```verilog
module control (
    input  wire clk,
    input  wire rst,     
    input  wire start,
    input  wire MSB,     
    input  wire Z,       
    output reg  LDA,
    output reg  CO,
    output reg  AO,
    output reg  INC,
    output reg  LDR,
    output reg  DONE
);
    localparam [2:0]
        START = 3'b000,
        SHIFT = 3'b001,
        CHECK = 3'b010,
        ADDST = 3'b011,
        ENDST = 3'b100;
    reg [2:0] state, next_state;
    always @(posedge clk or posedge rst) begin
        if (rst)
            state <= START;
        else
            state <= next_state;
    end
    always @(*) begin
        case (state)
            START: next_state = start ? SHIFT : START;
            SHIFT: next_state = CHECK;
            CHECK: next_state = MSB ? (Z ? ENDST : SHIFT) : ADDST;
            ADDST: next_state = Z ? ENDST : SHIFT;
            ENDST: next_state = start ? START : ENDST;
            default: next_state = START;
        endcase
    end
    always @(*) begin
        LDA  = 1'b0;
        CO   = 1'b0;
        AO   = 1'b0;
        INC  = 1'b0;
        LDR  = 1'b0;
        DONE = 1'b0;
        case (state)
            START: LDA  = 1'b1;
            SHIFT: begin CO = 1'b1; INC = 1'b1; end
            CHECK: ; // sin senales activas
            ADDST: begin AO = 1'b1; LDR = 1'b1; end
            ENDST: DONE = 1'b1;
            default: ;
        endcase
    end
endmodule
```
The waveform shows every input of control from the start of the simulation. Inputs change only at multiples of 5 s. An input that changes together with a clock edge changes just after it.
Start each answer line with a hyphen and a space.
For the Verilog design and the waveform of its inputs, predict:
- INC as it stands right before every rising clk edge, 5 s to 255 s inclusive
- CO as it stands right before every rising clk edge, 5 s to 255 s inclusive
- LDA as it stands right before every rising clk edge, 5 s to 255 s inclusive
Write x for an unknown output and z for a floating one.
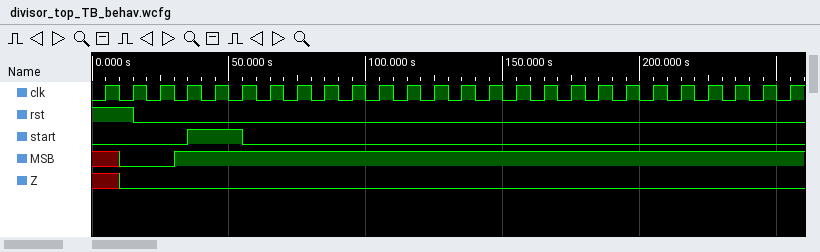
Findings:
- 0 0 0 0 0 1 0 1 0 1 0 1 0 1 0 1 0 1 0 1 0 1 0 1 0 1
- 0 0 0 0 0 1 0 1 0 1 0 1 0 1 0 1 0 1 0 1 0 1 0 1 0 1
- 1 1 1 1 1 0 0 0 0 0 0 0 0 0 0 0 0 0 0 0 0 0 0 0 0 0
